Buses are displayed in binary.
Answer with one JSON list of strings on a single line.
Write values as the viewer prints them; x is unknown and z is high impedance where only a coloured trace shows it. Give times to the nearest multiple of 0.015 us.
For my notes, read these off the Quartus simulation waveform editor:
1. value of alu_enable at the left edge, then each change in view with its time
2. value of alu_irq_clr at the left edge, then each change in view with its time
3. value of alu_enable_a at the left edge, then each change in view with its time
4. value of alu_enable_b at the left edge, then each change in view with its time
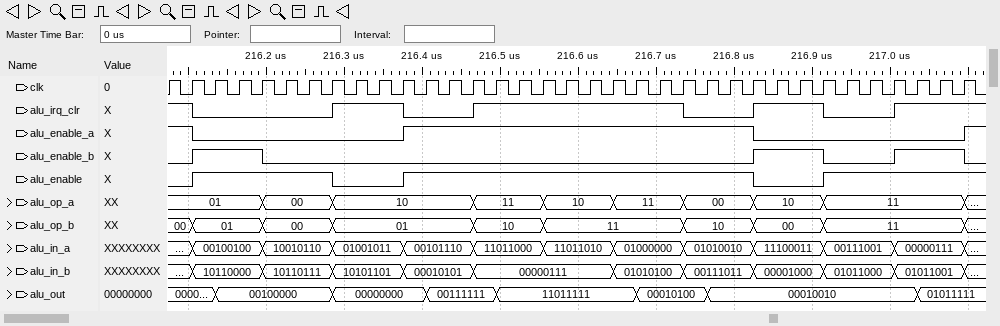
["0, 1 at 216.105 us, 0 at 216.285 us, 1 at 216.375 us, 0 at 216.825 us, 1 at 216.915 us", "1, 0 at 216.105 us, 1 at 216.285 us, 0 at 216.375 us, 1 at 216.465 us, 0 at 216.735 us, 1 at 216.825 us, 0 at 216.915 us, 1 at 217.005 us", "1, 0 at 216.105 us, 1 at 216.375 us, 0 at 216.825 us, 1 at 217.095 us", "0, 1 at 216.105 us, 0 at 216.195 us, 1 at 216.825 us, 0 at 216.915 us, 1 at 217.005 us, 0 at 217.095 us"]
